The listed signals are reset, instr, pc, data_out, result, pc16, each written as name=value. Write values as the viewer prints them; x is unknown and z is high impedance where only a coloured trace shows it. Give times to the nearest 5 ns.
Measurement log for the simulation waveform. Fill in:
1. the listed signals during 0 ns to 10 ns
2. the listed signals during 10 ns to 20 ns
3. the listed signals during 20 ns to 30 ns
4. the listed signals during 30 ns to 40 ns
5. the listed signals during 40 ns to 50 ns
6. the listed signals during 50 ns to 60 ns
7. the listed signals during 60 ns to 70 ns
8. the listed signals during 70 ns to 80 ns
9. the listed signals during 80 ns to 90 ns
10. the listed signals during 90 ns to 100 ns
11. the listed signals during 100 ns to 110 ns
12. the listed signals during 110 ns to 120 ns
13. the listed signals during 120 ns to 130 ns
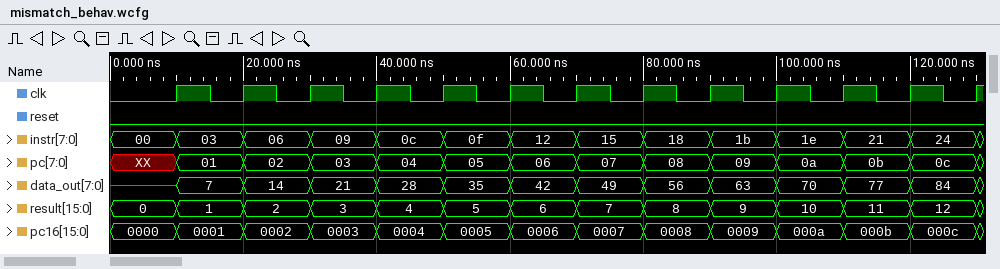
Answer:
reset=0, instr=00, pc=XX, data_out=z, result=0, pc16=0000
reset=0, instr=03, pc=01, data_out=7, result=1, pc16=0001
reset=0, instr=06, pc=02, data_out=14, result=2, pc16=0002
reset=0, instr=09, pc=03, data_out=21, result=3, pc16=0003
reset=0, instr=0c, pc=04, data_out=28, result=4, pc16=0004
reset=0, instr=0f, pc=05, data_out=35, result=5, pc16=0005
reset=0, instr=12, pc=06, data_out=42, result=6, pc16=0006
reset=0, instr=15, pc=07, data_out=49, result=7, pc16=0007
reset=0, instr=18, pc=08, data_out=56, result=8, pc16=0008
reset=0, instr=1b, pc=09, data_out=63, result=9, pc16=0009
reset=0, instr=1e, pc=0a, data_out=70, result=10, pc16=000a
reset=0, instr=21, pc=0b, data_out=77, result=11, pc16=000b
reset=0, instr=24, pc=0c, data_out=84, result=12, pc16=000c
